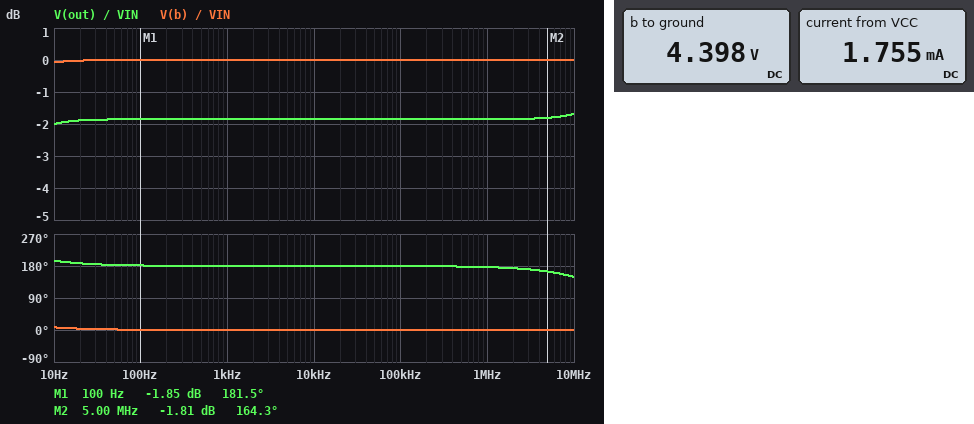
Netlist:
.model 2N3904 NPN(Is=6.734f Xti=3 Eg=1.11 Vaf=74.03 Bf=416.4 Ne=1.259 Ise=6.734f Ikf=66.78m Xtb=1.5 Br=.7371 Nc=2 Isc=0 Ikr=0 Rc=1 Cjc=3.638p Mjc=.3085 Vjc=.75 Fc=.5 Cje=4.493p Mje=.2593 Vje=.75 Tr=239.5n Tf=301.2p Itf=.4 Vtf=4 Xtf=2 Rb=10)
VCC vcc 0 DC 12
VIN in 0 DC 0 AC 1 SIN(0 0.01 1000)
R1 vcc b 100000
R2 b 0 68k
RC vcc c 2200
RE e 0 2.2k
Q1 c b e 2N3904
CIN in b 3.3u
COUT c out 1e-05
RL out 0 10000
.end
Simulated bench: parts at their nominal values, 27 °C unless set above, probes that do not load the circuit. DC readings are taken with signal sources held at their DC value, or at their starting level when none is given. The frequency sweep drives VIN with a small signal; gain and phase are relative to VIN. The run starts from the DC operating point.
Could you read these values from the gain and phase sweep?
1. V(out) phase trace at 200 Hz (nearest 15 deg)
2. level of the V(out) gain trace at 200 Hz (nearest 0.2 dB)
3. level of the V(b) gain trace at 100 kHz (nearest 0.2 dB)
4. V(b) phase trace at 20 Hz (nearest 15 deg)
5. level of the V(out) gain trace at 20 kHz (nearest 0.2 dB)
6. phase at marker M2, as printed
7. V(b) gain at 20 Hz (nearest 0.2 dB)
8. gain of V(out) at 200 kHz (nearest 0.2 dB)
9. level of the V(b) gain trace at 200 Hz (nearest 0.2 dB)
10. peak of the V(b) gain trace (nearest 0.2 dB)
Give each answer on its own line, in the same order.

180 deg
-1.8 dB
0 dB
0 deg
-1.8 dB
164.3 deg
0 dB
-1.8 dB
0 dB
0 dB
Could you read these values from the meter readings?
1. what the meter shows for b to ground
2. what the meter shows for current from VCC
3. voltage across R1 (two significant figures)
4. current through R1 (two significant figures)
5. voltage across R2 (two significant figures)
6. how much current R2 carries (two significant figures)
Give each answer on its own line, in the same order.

4.398 V
1.755 mA
7.6 V
76 µA
4.4 V
65 µA
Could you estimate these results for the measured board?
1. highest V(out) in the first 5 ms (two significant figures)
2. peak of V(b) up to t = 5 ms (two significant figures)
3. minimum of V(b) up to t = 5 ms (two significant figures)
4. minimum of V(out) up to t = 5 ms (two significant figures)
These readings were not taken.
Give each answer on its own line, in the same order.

8.1 mV
4.4 V
4.4 V
-8.1 mV
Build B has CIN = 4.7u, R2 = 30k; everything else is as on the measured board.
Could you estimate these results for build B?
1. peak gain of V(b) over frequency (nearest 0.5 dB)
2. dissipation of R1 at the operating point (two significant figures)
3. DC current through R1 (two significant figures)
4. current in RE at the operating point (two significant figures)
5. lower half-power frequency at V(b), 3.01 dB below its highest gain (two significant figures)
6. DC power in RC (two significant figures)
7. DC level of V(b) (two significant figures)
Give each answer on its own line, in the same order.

0 dB
880 µW
94 µA
890 µA
1.6 Hz
1.7 mW
2.6 V
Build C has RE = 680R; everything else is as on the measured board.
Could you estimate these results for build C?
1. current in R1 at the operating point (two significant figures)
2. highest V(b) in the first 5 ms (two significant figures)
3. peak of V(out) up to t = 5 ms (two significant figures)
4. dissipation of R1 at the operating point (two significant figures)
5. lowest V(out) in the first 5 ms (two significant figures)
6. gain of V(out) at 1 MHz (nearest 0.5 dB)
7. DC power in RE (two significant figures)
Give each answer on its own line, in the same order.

85 µA
3.5 V
20 mV
720 µW
-11 mV
3.0 dB
12 mW
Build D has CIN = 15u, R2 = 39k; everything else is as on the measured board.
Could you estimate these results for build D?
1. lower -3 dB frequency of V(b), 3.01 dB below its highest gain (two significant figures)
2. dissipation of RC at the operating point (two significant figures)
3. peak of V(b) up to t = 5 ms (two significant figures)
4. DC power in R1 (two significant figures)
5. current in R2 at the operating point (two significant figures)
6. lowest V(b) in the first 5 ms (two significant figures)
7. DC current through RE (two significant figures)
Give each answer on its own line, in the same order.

410 mHz
2.8 mW
3.2 V
780 µW
81 µA
3.1 V
1.1 mA
